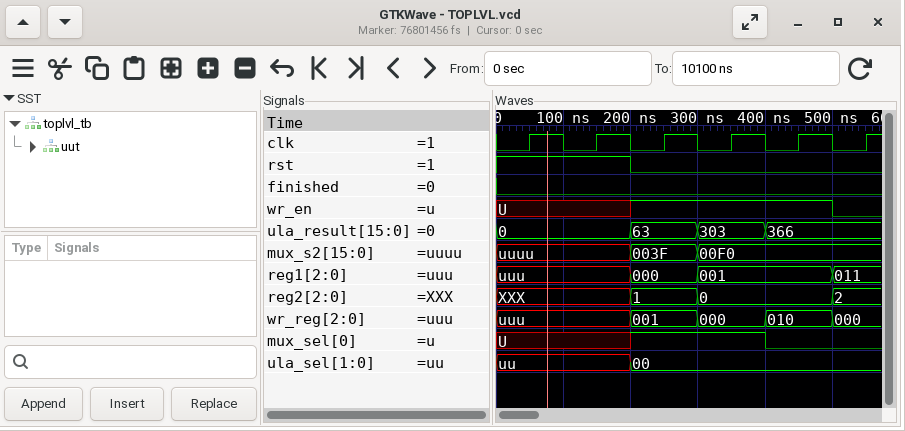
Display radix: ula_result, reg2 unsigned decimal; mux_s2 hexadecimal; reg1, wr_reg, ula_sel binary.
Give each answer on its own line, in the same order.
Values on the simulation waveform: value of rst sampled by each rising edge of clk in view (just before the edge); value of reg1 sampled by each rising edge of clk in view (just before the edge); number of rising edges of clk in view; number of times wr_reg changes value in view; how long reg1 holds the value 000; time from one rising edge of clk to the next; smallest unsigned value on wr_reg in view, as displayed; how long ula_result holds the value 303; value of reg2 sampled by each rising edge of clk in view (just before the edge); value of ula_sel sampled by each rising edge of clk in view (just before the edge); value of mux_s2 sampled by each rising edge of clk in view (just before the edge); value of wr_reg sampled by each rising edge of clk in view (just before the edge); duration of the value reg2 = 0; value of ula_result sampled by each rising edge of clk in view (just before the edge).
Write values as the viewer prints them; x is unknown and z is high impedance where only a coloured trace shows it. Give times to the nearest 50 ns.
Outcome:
1 1 0 0 0 0
uuu, uuu, 000, 001, 001, 011
6
4
100 ns
100 ns
000
100 ns
XXX, XXX, 1, 0, 0, 2
uu, uu, 00, 00, 00, 00
uuuu, uuuu, 003F, 00F0, 00F0, 00F0
uuu, uuu, 001, 000, 010, 000
200 ns
0, 0, 63, 303, 366, 366
